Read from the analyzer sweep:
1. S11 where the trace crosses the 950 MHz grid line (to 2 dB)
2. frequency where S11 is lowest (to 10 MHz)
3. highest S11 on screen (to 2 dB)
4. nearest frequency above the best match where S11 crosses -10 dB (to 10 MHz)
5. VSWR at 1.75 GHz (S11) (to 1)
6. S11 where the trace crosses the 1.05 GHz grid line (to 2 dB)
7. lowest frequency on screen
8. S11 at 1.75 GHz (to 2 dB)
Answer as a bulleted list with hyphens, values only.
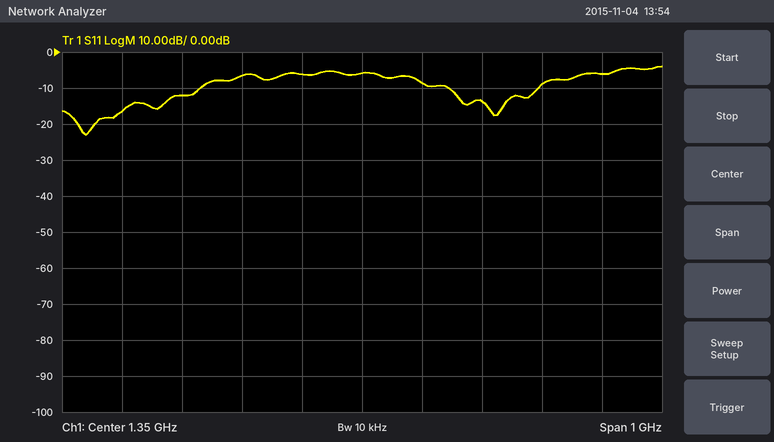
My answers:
- -16 dB
- 890 MHz
- -4 dB
- 1.08 GHz
- 3
- -12 dB
- 850 MHz
- -6 dB
